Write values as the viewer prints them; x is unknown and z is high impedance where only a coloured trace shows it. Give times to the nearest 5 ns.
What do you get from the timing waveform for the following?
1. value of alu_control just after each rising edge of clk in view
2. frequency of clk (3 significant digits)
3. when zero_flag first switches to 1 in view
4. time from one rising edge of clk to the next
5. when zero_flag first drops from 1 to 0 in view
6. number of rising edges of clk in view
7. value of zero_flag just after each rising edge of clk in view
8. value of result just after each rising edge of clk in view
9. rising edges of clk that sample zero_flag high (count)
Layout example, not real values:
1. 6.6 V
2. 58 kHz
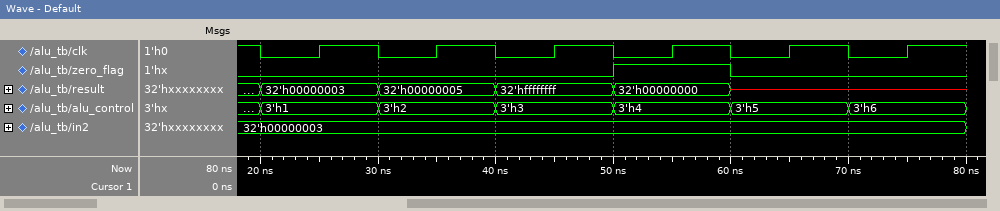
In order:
1. 3'h1, 3'h2, 3'h3, 3'h4, 3'h5, 3'h6
2. 100 MHz
3. 50 ns
4. 10 ns
5. 60 ns
6. 6
7. 0 0 0 1 0 0
8. 32'h00000003, 32'h00000005, 32'hffffffff, 32'h00000000, x, x
9. 1
